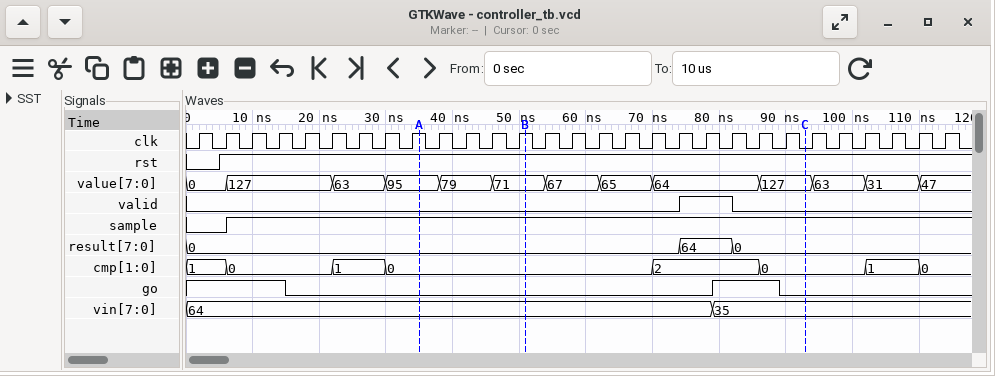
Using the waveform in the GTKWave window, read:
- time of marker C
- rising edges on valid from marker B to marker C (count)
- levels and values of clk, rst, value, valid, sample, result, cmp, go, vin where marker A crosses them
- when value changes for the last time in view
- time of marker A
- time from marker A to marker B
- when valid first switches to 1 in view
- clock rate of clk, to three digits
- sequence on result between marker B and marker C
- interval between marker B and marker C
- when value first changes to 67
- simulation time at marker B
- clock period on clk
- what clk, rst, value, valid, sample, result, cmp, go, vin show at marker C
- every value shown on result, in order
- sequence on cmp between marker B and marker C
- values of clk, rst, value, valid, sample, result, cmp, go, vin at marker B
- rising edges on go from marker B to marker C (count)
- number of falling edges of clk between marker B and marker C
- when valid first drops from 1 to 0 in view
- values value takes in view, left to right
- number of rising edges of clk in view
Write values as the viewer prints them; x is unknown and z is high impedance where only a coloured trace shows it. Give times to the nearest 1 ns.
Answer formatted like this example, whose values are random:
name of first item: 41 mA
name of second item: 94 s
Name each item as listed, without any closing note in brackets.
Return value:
time of marker C: 93 ns
rising edges on valid from marker B to marker C: 1
levels and values of clk, rst, value, valid, sample, result, cmp, go, vin where marker A crosses them: clk=1, rst=1, value=95, valid=0, sample=1, result=0, cmp=0, go=0, vin=64
when value changes for the last time in view: 110 ns
time of marker A: 35 ns
time from marker A to marker B: 16 ns
when valid first switches to 1 in view: 74 ns
clock rate of clk, to three digits: 250 MHz
sequence on result between marker B and marker C: 0, 64, 0
interval between marker B and marker C: 42 ns
when value first changes to 67: 54 ns
simulation time at marker B: 51 ns
clock period on clk: 4 ns
what clk, rst, value, valid, sample, result, cmp, go, vin show at marker C: clk=0, rst=1, value=127, valid=0, sample=1, result=0, cmp=0, go=0, vin=35
every value shown on result, in order: 0, 64, 0
sequence on cmp between marker B and marker C: 0, 2, 0
values of clk, rst, value, valid, sample, result, cmp, go, vin at marker B: clk=1, rst=1, value=71, valid=0, sample=1, result=0, cmp=0, go=0, vin=64
rising edges on go from marker B to marker C: 1
number of falling edges of clk between marker B and marker C: 11
when valid first drops from 1 to 0 in view: 82 ns
values value takes in view, left to right: 0, 127, 63, 95, 79, 71, 67, 65, 64, 127, 63, 31, 47
number of rising edges of clk in view: 29
